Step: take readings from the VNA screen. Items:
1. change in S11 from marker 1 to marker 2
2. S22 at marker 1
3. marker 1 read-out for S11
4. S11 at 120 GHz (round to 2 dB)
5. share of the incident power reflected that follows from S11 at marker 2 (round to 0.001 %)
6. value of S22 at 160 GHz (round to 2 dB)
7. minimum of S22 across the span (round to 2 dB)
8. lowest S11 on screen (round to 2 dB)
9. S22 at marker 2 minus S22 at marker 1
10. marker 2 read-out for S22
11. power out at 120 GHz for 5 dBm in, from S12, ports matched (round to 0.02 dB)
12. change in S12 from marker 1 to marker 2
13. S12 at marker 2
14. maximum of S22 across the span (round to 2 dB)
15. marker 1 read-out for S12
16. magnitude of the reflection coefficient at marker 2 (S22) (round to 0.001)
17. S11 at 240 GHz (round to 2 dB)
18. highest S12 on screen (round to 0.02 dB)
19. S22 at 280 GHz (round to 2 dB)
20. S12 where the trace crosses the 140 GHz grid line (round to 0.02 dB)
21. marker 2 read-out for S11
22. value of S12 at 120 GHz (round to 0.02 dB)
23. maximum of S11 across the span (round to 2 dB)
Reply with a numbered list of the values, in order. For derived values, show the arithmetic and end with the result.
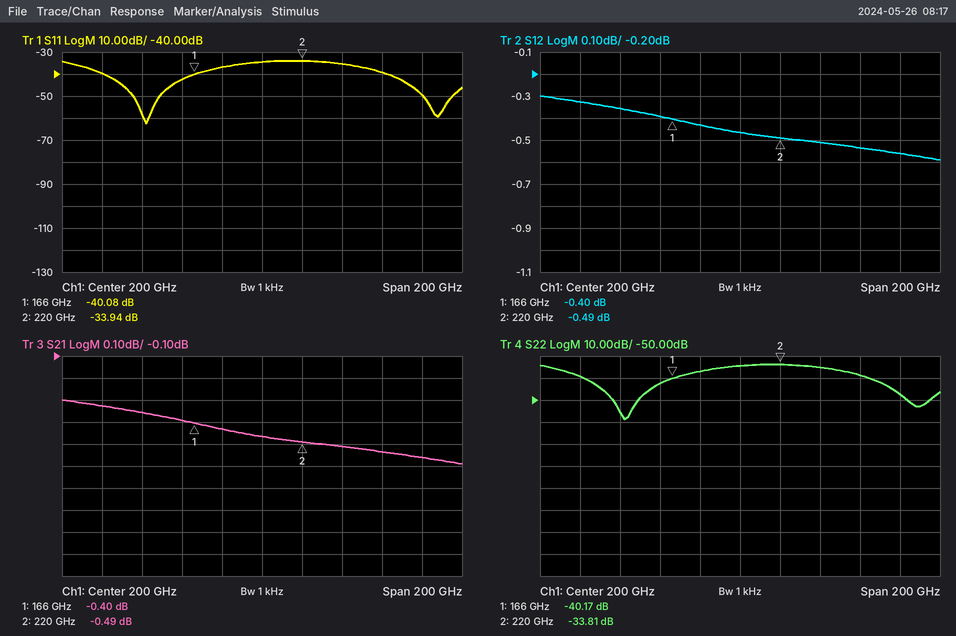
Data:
1. -33.94 − (-40.08) = 6.14 dB
2. -40.17 dB
3. -40.08 dB
4. -40 dB
5. 10^(-33.94/10) ≈ 0.040 %
6. -42 dB
7. -58 dB
8. -62 dB
9. -33.81 − (-40.17) = 6.36 dB
10. -33.81 dB
11. 5 dBm + (-0.32 dB) = 4.68 dBm
12. -0.49 − (-0.4) = -0.09 dB
13. -0.49 dB
14. -34 dB
15. -0.40 dB
16. 10^(-33.81/20) ≈ 0.020
17. -36 dB
18. -0.30 dB
19. -48 dB
20. -0.36 dB
21. -33.94 dB
22. -0.32 dB
23. -34 dB
